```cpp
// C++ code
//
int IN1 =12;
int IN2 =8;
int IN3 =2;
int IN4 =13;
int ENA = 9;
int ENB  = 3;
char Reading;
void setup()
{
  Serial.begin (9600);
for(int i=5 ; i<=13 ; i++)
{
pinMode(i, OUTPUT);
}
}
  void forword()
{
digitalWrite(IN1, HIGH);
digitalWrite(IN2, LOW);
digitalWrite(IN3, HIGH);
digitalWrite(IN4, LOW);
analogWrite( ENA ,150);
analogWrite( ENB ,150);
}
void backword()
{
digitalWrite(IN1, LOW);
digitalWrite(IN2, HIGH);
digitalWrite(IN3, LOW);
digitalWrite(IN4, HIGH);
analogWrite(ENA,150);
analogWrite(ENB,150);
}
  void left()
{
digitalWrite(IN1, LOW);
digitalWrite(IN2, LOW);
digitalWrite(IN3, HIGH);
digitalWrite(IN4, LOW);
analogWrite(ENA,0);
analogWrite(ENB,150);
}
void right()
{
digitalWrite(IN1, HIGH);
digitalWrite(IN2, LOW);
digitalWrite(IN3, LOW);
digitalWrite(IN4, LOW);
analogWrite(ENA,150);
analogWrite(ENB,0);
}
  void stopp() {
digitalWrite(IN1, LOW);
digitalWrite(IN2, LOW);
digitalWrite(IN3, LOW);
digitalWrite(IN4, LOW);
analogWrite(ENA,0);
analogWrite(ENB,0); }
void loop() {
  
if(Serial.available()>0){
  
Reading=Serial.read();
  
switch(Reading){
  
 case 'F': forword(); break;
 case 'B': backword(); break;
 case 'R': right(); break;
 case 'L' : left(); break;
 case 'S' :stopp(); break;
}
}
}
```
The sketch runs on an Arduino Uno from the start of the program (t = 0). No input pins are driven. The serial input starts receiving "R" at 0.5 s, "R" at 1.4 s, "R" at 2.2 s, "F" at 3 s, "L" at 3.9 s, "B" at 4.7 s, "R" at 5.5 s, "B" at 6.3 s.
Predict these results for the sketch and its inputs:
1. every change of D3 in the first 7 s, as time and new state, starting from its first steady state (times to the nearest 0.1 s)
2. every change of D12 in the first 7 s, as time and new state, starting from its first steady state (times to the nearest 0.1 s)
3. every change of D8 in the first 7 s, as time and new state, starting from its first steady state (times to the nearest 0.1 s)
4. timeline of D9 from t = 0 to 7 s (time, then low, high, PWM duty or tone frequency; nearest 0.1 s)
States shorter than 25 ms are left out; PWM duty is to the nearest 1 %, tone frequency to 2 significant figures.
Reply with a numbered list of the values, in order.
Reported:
1. 0.5 s low; 3 s PWM 59 %; 5.5 s low; 6.3 s PWM 59 %
2. 0 s low; 0.5 s high; 3.9 s low; 5.5 s high; 6.3 s low
3. 0 s low; 4.7 s high; 5.5 s low; 6.3 s high
4. 0 s low; 0.5 s PWM 59 %; 3.9 s low; 4.7 s PWM 59 %
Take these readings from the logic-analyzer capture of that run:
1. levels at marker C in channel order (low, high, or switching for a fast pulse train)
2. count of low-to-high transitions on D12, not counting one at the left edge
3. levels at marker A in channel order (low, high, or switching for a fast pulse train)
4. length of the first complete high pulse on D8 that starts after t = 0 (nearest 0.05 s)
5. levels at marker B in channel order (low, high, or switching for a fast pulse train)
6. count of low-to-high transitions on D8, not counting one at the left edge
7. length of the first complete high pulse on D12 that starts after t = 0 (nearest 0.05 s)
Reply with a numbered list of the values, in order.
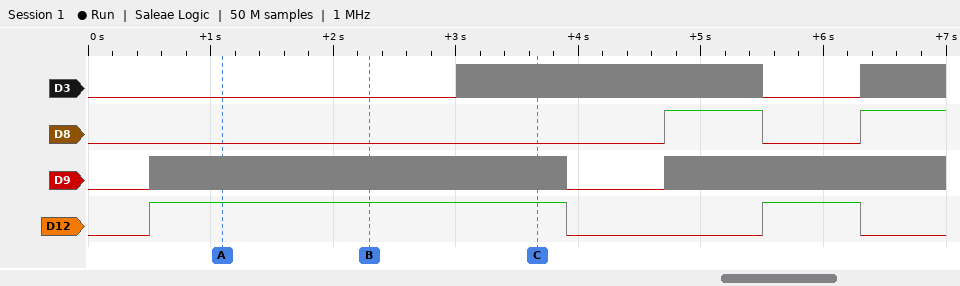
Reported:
1. D3 switching, D8 low, D9 switching, D12 high
2. 2
3. D3 low, D8 low, D9 switching, D12 high
4. 0.80 s
5. D3 low, D8 low, D9 switching, D12 high
6. 2
7. 3.40 s
